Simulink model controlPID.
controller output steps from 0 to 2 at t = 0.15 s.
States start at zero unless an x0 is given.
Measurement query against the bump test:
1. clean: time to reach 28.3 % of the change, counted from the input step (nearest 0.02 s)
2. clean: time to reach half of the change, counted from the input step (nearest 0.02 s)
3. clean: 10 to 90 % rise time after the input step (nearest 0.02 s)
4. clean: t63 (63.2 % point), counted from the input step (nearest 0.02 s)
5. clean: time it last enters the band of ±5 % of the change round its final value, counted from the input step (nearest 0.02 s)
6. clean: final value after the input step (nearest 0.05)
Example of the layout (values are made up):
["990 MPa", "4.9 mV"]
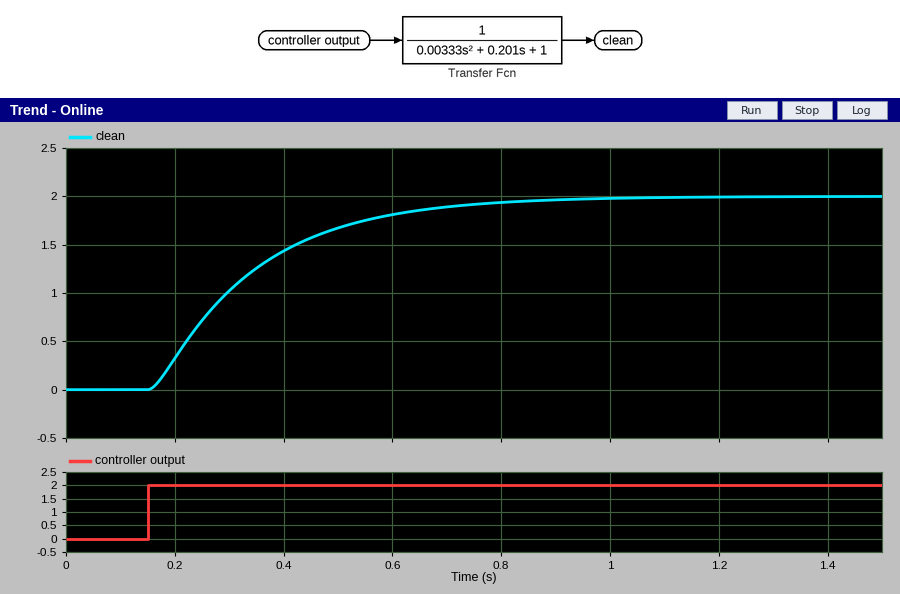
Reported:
["0.08 s", "0.14 s", "0.40 s", "0.20 s", "0.56 s", "2.00"]
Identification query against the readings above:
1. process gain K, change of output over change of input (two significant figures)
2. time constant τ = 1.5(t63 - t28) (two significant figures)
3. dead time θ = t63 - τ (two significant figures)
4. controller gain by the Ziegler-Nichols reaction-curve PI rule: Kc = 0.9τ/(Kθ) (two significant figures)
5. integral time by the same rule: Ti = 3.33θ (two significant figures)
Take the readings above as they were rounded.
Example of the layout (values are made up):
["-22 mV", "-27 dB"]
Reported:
["1.0", "0.18 s", "0.020 s", "8.1", "0.067 s"]
